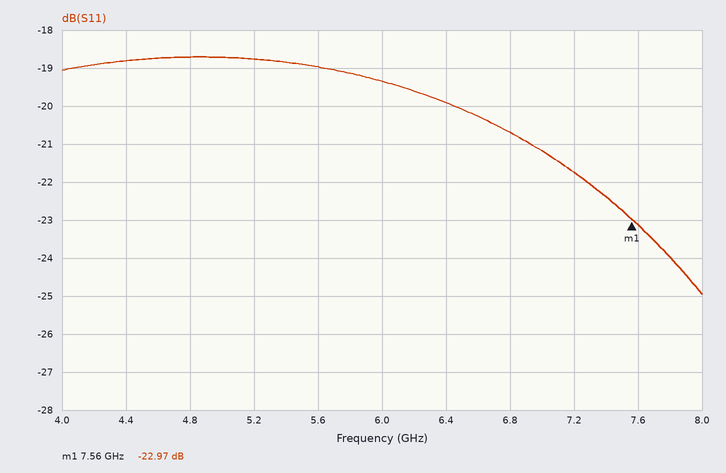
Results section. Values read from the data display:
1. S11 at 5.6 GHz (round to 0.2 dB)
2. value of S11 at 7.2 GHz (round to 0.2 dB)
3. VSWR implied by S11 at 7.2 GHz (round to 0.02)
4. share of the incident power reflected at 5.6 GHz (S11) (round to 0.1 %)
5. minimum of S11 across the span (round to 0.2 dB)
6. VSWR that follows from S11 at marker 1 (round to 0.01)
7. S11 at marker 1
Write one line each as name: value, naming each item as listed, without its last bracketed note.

S11 at 5.6 GHz: -19.0 dB
value of S11 at 7.2 GHz: -21.8 dB
VSWR implied by S11 at 7.2 GHz: 1.18
share of the incident power reflected at 5.6 GHz (S11): 1.3 %
minimum of S11 across the span: -25.0 dB
VSWR that follows from S11 at marker 1: 1.15
S11 at marker 1: -22.97 dB
